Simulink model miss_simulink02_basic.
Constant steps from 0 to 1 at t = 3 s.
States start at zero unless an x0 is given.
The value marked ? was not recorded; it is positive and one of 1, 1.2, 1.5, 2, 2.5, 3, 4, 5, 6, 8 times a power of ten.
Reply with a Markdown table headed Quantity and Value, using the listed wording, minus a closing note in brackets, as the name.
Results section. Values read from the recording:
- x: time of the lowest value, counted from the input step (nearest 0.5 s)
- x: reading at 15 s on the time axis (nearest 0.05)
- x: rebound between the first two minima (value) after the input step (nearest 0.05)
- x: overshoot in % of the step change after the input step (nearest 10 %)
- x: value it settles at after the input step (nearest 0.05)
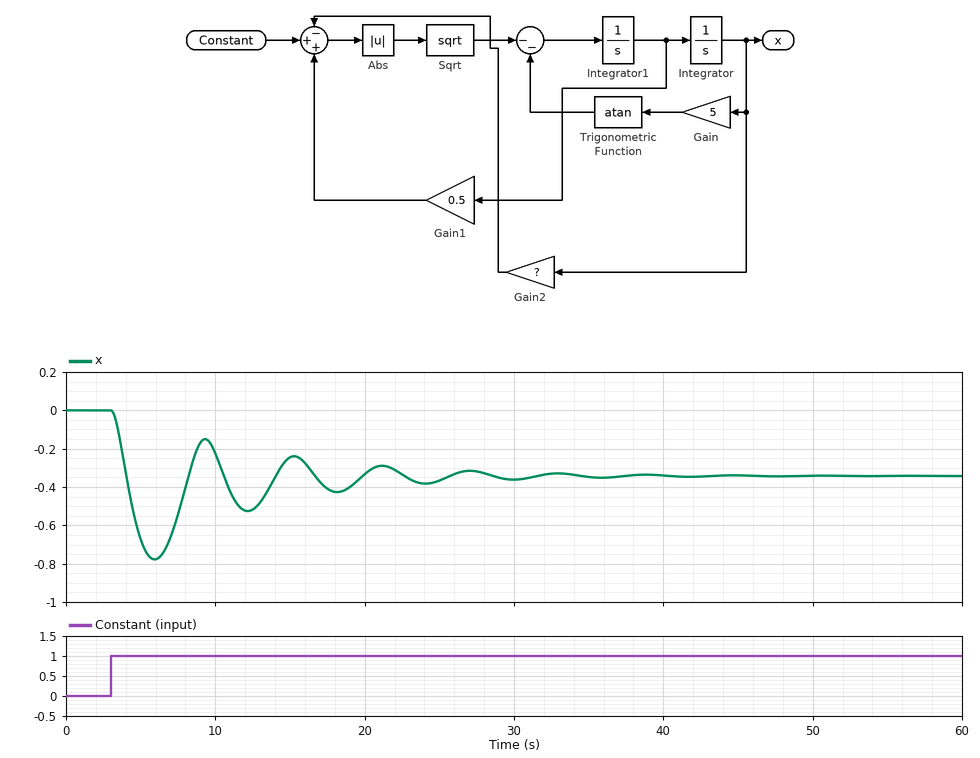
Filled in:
| Quantity | Value |
|---|---|
| x: time of the lowest value, counted from the input step | 3.0 s |
| x: reading at 15 s on the time axis | -0.25 |
| x: rebound between the first two minima (value) after the input step | -0.15 |
| x: overshoot in % of the step change after the input step | 130 % |
| x: value it settles at after the input step | -0.35 |
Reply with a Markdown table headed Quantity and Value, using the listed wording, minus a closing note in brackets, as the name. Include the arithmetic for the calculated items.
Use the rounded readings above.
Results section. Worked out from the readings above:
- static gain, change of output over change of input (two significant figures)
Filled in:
| Quantity | Value |
|---|---|
| static gain, change of output over change of input | (-0.35 - 0) / (1 - 0) = -0.35 |
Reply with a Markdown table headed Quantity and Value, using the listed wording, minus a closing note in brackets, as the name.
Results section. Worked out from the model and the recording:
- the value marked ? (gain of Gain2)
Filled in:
| Quantity | Value |
|---|---|
| the value marked ? | 0.25 |
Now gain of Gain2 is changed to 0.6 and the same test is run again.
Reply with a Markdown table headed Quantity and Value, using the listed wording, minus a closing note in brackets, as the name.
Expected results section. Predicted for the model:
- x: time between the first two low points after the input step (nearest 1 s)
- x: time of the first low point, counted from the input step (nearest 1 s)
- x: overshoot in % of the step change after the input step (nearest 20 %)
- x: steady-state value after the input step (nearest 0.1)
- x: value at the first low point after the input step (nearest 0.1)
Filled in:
| Quantity | Value |
|---|---|
| x: time between the first two low points after the input step | 9 s |
| x: time of the first low point, counted from the input step | 4 s |
| x: overshoot in % of the step change after the input step | 160 % |
| x: steady-state value after the input step | -0.4 |
| x: value at the first low point after the input step | -1.1 |
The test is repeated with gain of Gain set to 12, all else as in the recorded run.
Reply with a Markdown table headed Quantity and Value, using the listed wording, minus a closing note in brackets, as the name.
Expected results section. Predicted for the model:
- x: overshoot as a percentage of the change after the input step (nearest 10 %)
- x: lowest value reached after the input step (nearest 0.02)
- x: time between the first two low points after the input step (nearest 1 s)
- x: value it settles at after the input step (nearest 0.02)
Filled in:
| Quantity | Value |
|---|---|
| x: overshoot as a percentage of the change after the input step | 140 % |
| x: lowest value reached after the input step | -0.32 |
| x: time between the first two low points after the input step | 4 s |
| x: value it settles at after the input step | -0.14 |
